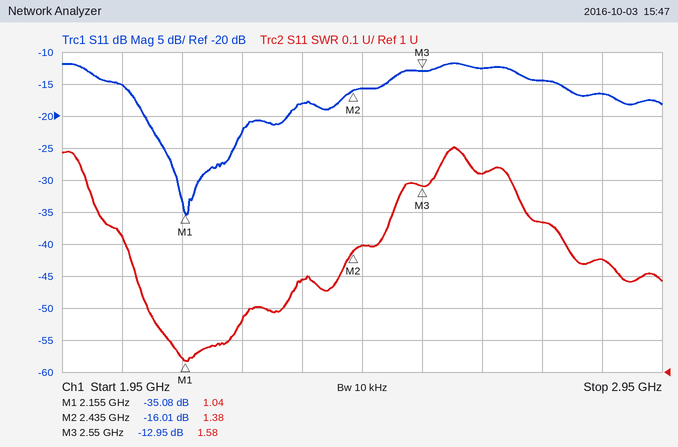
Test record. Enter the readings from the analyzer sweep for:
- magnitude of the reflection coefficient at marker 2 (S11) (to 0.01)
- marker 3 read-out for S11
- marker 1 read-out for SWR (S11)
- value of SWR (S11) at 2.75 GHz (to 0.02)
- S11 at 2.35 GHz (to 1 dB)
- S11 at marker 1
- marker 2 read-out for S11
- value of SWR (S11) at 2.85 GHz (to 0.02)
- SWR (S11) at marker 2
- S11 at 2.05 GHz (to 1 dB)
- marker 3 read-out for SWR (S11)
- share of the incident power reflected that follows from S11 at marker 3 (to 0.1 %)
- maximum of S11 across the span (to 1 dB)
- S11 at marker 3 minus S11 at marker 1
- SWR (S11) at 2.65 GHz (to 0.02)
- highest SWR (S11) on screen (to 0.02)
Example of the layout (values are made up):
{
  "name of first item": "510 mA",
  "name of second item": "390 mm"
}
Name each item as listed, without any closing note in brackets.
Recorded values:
{
  "magnitude of the reflection coefficient at marker 2 (S11)": "0.16",
  "marker 3 read-out for S11": "-12.95 dB",
  "marker 1 read-out for SWR": "1.04",
  "value of SWR (S11) at 2.75 GHz": "1.46",
  "S11 at 2.35 GHz": "-18 dB",
  "S11 at marker 1": "-35.08 dB",
  "marker 2 read-out for S11": "-16.01 dB",
  "value of SWR (S11) at 2.85 GHz": "1.36",
  "SWR (S11) at marker 2": "1.38",
  "S11 at 2.05 GHz": "-15 dB",
  "marker 3 read-out for SWR": "1.58",
  "share of the incident power reflected that follows from S11 at marker 3": "5.1 %",
  "maximum of S11 across the span": "-12 dB",
  "S11 at marker 3 minus S11 at marker 1": "22.13 dB",
  "SWR (S11) at 2.65 GHz": "1.62",
  "highest SWR (S11) on screen": "1.70"
}
